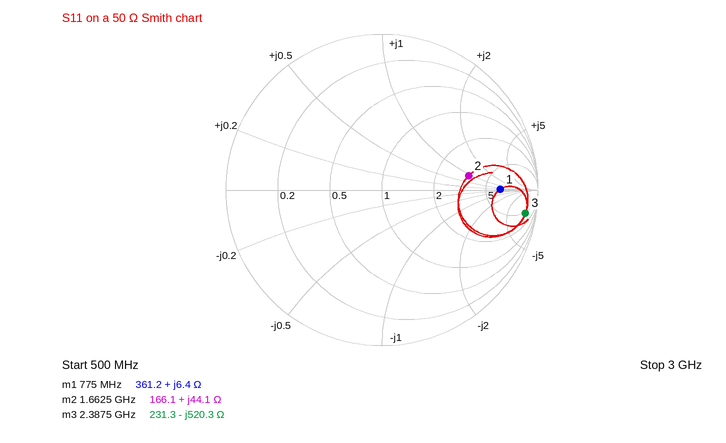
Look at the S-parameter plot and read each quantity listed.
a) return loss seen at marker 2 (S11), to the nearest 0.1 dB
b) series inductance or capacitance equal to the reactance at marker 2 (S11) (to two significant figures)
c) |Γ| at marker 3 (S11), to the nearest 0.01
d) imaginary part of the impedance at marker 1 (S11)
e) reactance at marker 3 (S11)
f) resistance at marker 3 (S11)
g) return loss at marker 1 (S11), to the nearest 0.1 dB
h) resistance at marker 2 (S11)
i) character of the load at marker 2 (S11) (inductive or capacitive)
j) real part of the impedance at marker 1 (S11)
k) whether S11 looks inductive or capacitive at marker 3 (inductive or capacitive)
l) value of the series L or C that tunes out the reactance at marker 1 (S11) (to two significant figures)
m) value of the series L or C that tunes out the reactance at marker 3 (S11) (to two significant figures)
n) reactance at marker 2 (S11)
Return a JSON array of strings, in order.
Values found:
["5.0 dB", "4.2 nH", "0.93", "+6.4 Ω", "-520.3 Ω", "231.3 Ω", "2.4 dB", "166.1 Ω", "inductive", "361.2 Ω", "capacitive", "32 pF", "35 nH", "+44.1 Ω"]
